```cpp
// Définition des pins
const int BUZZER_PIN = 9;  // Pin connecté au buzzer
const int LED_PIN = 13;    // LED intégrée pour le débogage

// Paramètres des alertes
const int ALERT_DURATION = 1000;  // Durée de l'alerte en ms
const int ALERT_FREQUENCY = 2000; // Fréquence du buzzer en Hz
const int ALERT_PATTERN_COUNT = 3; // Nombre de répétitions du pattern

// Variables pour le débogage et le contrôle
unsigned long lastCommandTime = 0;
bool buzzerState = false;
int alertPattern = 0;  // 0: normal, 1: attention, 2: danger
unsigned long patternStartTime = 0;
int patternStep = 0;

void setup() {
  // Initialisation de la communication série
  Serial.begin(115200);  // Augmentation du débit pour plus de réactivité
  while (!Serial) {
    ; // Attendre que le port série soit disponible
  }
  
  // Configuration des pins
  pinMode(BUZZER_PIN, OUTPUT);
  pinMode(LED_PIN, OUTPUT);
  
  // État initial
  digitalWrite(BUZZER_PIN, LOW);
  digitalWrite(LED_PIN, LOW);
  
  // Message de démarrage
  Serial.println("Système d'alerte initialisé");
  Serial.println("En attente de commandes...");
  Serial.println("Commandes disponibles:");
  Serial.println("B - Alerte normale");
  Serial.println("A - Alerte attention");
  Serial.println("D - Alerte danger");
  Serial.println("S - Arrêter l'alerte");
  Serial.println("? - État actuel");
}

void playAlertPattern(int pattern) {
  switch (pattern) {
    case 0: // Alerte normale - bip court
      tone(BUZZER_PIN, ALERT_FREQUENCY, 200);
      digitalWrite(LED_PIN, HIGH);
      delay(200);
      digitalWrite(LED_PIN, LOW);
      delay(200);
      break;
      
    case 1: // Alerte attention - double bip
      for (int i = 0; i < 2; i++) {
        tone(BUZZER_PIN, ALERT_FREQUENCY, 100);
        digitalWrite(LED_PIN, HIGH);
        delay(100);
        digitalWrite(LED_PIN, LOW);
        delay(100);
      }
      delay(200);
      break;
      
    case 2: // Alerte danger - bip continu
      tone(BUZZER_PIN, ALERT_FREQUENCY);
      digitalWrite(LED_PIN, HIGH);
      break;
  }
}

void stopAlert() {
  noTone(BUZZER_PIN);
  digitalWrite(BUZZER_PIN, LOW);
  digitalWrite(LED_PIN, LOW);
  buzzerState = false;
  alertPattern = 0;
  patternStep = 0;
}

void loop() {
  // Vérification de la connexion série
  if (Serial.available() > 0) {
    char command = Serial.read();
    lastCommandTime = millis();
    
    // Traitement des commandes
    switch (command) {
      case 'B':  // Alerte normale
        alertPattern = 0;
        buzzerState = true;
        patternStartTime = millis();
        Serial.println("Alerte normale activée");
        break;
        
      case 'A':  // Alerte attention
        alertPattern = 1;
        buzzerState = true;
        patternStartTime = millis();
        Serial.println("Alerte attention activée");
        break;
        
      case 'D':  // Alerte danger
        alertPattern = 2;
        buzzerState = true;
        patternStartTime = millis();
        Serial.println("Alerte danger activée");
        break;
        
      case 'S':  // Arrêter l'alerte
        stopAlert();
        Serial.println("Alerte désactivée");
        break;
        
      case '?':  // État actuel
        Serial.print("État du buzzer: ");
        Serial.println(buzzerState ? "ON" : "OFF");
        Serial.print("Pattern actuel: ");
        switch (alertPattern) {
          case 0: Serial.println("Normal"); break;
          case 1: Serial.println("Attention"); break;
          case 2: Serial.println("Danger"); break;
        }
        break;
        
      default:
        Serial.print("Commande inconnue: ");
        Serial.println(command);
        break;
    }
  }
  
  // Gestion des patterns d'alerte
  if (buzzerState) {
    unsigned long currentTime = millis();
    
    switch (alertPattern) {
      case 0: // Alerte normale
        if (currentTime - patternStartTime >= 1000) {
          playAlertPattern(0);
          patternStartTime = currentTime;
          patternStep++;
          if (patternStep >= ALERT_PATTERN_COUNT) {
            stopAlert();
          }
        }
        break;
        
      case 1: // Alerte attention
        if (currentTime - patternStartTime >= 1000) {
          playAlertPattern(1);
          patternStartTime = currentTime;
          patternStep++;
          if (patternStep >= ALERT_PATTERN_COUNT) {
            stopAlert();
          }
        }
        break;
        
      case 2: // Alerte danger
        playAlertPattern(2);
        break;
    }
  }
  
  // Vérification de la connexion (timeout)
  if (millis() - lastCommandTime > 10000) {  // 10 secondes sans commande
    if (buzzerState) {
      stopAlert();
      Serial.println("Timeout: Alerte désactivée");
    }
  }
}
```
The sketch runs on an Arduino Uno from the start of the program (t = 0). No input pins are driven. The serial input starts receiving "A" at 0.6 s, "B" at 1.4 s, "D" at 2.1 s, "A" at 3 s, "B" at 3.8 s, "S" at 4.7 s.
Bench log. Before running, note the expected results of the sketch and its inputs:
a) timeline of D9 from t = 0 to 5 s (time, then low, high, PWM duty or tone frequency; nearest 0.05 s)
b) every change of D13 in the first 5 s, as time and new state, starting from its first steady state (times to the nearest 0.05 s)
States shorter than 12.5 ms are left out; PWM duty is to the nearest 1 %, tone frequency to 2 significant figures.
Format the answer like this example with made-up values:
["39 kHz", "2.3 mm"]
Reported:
["0 s low; 2.1 s tone 2000 Hz; 4.7 s low", "0 s low; 2.1 s high; 4.7 s low"]
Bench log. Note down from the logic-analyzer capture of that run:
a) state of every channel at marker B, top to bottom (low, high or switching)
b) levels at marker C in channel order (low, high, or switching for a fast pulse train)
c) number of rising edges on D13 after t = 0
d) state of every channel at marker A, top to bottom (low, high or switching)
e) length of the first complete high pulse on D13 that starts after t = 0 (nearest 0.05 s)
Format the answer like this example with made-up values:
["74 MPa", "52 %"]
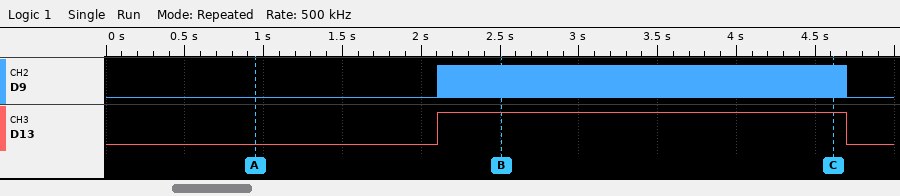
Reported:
["D9 switching, D13 high", "D9 switching, D13 high", "1", "D9 low, D13 low", "2.60 s"]
